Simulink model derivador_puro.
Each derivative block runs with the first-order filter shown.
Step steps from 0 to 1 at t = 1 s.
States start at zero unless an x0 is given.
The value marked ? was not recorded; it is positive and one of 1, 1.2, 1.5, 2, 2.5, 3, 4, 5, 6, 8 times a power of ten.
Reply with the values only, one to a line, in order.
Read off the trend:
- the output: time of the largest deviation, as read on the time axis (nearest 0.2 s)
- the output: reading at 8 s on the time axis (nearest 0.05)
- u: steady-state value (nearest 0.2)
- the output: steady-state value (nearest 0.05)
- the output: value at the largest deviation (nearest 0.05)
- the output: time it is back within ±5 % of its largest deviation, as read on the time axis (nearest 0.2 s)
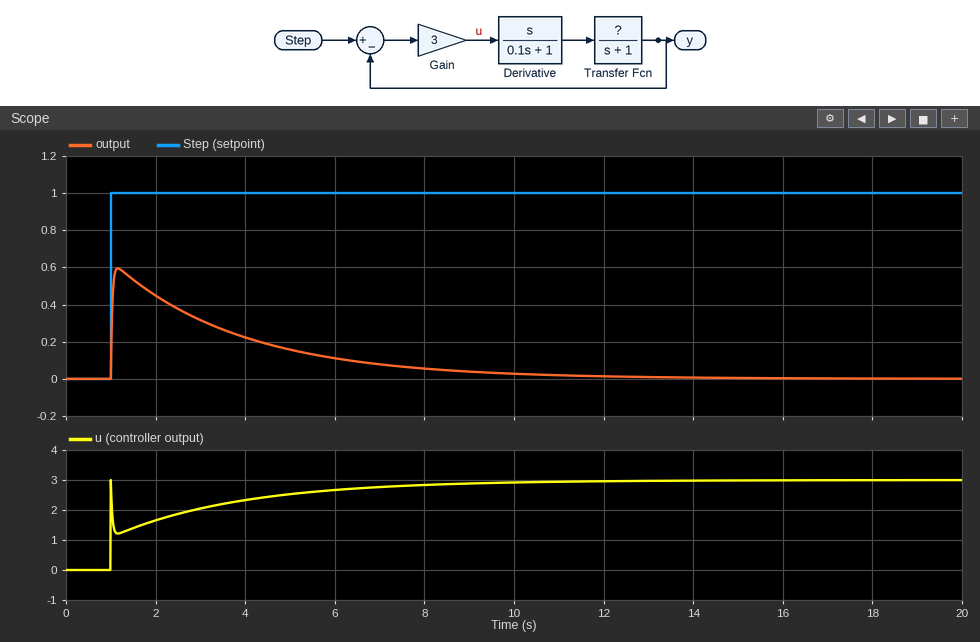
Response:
1.2 s
0.05
3.0
0.00
0.60
9.8 s
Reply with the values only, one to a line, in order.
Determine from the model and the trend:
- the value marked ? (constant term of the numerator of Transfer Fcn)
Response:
0.6
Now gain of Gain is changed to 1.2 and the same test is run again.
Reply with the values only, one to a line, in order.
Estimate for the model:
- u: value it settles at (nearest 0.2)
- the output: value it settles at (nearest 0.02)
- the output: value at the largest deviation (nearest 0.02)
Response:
1.2
0.00
0.36
